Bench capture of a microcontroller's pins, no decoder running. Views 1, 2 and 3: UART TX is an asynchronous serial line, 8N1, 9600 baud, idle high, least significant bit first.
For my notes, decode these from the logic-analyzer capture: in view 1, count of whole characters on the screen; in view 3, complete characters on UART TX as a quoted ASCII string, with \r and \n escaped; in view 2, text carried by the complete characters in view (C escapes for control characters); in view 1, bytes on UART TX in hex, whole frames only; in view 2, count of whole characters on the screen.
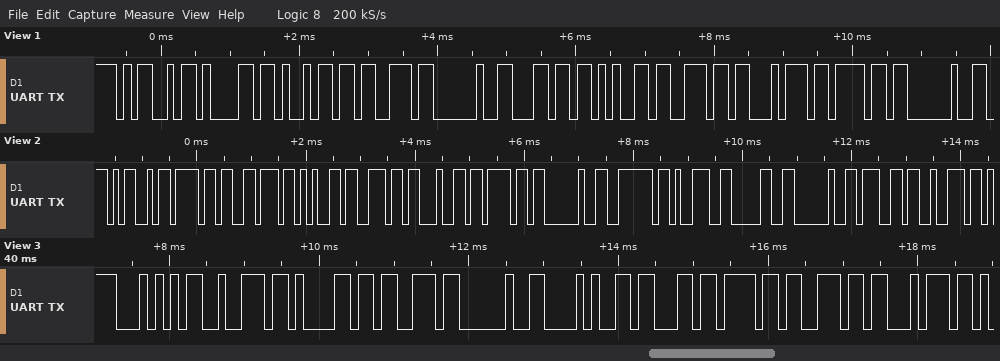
11
"Tras (cont"
"Movendo ~90 gr"
0x4D 0x61 0x69 0x73 0x20 0x6C 0x65 0x6E 0x74 0x6F 0x20
14
